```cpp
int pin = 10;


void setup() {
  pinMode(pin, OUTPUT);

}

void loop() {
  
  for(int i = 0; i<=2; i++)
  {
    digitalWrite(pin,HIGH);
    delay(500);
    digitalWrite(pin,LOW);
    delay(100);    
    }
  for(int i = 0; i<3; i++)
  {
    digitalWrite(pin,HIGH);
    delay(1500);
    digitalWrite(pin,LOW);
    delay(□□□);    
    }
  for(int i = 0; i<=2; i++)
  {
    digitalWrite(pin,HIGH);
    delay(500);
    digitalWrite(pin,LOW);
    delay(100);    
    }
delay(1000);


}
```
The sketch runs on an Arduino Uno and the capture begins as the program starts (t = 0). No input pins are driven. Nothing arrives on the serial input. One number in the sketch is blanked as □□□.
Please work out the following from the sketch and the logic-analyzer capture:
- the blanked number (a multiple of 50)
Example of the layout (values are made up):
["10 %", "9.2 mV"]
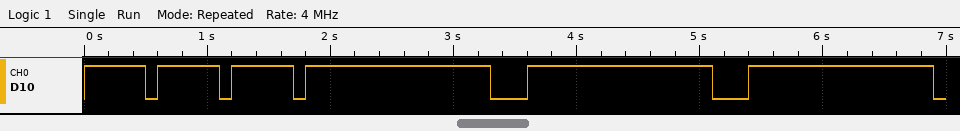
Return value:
["300"]
